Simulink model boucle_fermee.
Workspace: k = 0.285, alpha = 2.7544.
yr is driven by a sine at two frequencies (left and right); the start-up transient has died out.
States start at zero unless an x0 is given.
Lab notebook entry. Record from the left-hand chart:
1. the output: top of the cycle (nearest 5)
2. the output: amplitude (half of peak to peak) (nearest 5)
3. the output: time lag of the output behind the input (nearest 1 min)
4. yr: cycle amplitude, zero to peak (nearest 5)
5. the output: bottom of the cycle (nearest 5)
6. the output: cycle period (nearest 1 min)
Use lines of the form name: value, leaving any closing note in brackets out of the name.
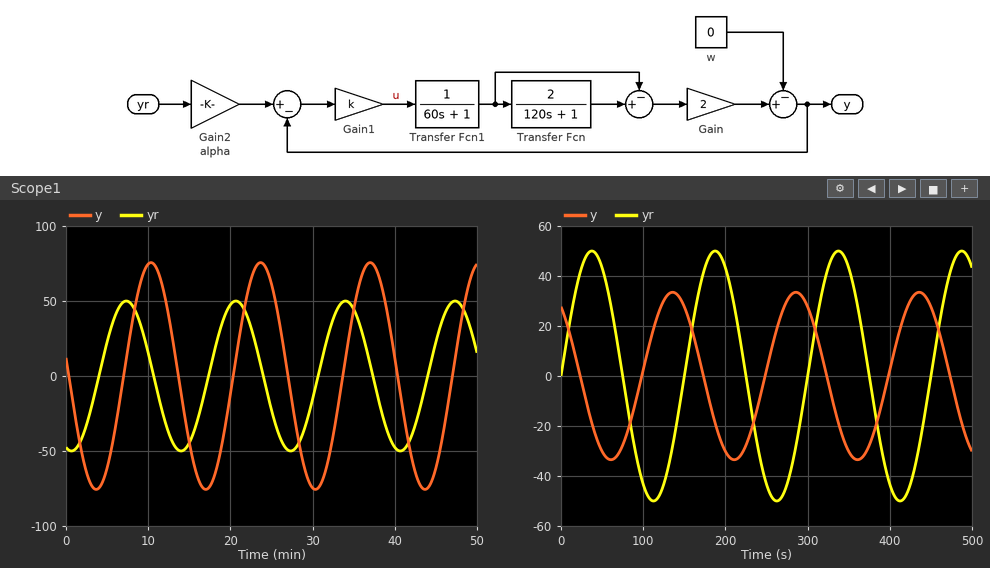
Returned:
the output: top of the cycle: 75
the output: amplitude (half of peak to peak): 75
the output: time lag of the output behind the input: 3 min
yr: cycle amplitude, zero to peak: 50
the output: bottom of the cycle: -75
the output: cycle period: 13 min
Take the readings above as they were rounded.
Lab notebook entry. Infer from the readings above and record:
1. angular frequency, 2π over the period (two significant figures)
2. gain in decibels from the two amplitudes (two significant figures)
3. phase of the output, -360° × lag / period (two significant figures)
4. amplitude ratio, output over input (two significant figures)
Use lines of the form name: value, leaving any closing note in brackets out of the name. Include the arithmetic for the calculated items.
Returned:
angular frequency, 2π over the period: 2π / 13 = 0.48 rad/min
gain in decibels from the two amplitudes: 20 log10(75 / 50) = 3.5 dB
phase of the output, -360° × lag / period: -360 × 3 / 13 = -83°
amplitude ratio, output over input: 75 / 50 = 1.5
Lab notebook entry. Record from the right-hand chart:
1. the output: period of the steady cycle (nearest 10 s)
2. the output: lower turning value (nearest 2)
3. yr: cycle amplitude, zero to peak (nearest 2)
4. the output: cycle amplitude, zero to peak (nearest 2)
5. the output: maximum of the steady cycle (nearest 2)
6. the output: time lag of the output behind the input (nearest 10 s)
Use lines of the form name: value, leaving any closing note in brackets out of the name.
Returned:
the output: period of the steady cycle: 150 s
the output: lower turning value: -34
yr: cycle amplitude, zero to peak: 50
the output: cycle amplitude, zero to peak: 34
the output: maximum of the steady cycle: 34
the output: time lag of the output behind the input: 100 s
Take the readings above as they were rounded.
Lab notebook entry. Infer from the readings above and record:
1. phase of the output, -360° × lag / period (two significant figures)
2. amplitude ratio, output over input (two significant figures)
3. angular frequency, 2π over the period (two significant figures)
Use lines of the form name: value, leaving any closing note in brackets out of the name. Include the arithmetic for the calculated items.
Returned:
phase of the output, -360° × lag / period: -360 × 100 / 150 = -240°
amplitude ratio, output over input: 34 / 50 = 0.68
angular frequency, 2π over the period: 2π / 150 = 0.042 rad/s
